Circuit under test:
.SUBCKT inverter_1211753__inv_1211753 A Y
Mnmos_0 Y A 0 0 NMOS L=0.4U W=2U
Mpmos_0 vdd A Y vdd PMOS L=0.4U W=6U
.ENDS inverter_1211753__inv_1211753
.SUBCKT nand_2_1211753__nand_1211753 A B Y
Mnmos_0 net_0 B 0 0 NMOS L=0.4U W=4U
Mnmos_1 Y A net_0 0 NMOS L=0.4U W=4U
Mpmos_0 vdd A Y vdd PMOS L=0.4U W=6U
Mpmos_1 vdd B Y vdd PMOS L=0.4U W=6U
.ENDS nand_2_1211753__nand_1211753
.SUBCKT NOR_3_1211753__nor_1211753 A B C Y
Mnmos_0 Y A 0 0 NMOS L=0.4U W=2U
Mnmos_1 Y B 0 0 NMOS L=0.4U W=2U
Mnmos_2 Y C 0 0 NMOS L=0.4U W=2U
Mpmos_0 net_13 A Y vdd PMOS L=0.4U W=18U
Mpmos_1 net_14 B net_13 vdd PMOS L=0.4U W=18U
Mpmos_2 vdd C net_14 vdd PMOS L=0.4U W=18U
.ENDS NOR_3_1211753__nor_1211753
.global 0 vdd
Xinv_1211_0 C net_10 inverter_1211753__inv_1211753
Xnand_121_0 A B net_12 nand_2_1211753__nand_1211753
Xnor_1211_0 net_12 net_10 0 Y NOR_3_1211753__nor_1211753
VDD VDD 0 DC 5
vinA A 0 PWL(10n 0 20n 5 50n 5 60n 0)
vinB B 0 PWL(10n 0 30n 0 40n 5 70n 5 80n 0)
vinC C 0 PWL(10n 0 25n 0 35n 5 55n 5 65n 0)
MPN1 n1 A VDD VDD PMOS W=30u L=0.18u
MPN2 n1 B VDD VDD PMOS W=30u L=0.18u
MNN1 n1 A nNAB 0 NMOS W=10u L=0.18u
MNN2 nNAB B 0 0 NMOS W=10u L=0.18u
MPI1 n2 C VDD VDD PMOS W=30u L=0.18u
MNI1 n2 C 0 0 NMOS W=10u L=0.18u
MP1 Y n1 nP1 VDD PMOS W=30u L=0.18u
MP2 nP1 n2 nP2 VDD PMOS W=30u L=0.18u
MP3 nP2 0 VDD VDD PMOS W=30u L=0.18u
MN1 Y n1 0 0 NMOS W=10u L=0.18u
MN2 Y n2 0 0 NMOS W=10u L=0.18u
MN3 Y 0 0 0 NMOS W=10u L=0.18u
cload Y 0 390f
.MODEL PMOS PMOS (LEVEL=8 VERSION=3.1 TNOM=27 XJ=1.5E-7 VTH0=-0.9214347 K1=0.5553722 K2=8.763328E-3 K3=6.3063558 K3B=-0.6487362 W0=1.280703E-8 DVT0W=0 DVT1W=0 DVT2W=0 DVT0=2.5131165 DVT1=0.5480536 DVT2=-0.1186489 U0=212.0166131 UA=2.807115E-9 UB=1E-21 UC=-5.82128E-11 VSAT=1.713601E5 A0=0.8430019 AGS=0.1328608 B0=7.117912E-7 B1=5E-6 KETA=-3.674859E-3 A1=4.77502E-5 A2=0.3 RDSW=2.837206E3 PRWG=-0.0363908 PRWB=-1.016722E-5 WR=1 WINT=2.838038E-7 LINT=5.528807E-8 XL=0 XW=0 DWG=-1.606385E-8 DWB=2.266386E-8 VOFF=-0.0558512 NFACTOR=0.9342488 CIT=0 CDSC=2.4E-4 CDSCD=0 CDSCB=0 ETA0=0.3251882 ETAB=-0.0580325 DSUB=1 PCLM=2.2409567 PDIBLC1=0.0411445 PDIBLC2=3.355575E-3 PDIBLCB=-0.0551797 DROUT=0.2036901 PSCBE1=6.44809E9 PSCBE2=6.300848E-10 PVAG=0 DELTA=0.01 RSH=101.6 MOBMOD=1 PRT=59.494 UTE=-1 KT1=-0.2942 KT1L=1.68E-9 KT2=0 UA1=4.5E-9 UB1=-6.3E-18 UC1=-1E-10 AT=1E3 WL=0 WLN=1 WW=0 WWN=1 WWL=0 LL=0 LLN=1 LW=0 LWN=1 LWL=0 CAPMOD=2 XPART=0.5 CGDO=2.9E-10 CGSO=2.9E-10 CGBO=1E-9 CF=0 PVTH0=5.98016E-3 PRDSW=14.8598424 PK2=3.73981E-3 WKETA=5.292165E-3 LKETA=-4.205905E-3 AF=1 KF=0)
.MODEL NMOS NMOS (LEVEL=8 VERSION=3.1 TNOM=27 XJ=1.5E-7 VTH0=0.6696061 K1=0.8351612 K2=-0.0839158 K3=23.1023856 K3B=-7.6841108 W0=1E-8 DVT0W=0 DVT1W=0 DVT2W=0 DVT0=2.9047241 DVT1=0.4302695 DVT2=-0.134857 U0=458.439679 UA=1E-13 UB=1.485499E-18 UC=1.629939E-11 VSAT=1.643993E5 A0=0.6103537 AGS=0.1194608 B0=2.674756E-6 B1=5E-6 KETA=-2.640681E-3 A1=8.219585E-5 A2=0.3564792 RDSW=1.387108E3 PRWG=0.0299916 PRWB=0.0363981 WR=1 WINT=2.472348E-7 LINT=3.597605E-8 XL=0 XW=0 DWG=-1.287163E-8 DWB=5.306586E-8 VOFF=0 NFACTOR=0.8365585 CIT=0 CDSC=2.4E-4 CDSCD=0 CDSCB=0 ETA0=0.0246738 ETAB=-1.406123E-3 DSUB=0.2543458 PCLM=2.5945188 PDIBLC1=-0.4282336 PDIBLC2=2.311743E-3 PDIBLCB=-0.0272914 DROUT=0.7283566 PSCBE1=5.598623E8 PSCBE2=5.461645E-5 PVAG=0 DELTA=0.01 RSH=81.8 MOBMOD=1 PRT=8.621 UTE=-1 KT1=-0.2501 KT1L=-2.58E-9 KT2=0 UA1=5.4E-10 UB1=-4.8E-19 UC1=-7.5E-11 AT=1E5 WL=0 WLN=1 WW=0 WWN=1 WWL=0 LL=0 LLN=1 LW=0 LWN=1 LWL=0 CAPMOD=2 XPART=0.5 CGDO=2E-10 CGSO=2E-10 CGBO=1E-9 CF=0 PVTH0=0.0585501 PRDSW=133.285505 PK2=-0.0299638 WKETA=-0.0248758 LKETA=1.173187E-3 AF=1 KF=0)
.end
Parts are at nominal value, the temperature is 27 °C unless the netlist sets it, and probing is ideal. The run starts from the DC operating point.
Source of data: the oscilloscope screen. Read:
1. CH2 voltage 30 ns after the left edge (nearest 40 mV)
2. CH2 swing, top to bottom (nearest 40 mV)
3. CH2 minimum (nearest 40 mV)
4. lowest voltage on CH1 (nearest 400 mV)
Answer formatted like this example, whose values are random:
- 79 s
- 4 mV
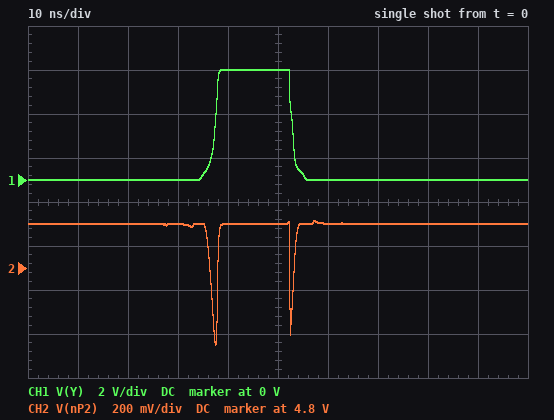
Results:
- 5.00 V
- 560 mV
- 4.44 V
- 0 V
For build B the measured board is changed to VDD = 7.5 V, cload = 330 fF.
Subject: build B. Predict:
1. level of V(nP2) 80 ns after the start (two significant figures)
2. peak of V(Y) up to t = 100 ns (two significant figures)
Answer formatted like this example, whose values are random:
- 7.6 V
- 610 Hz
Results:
- 7.5 V
- 190 mV
